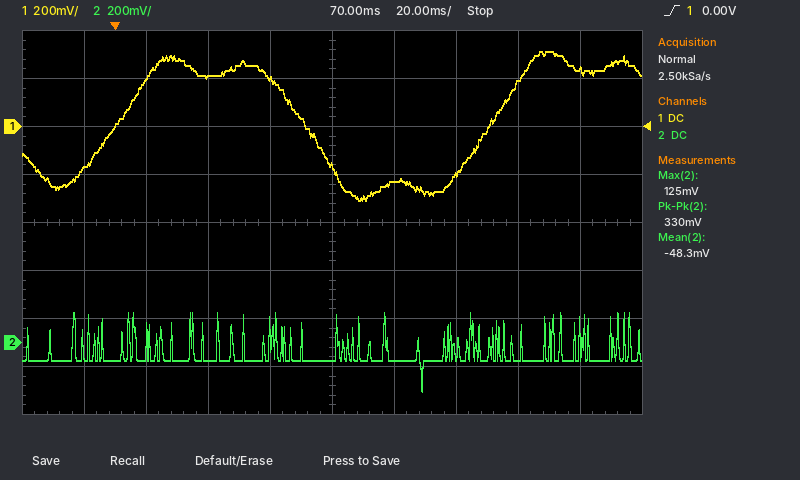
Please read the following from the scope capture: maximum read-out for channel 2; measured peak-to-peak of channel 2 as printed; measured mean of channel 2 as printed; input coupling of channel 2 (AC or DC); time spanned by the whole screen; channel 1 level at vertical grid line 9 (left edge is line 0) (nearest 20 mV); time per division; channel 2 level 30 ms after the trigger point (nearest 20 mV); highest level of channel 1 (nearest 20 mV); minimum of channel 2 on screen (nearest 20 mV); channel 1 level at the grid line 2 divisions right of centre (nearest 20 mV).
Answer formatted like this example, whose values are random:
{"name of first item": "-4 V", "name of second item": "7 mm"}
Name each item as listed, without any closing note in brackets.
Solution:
{"maximum read-out for channel 2": "125 mV", "measured peak-to-peak of channel 2 as printed": "330 mV", "measured mean of channel 2 as printed": "-48.3 mV", "input coupling of channel 2": "DC", "time spanned by the whole screen": "200 ms", "channel 1 level at vertical grid line 9 (left edge is line 0)": "240 mV", "time per division": "20 ms", "channel 2 level 30 ms after the trigger point": "-80 mV", "highest level of channel 1": "320 mV", "minimum of channel 2 on screen": "-200 mV", "channel 1 level at the grid line 2 divisions right of centre": "-200 mV"}
